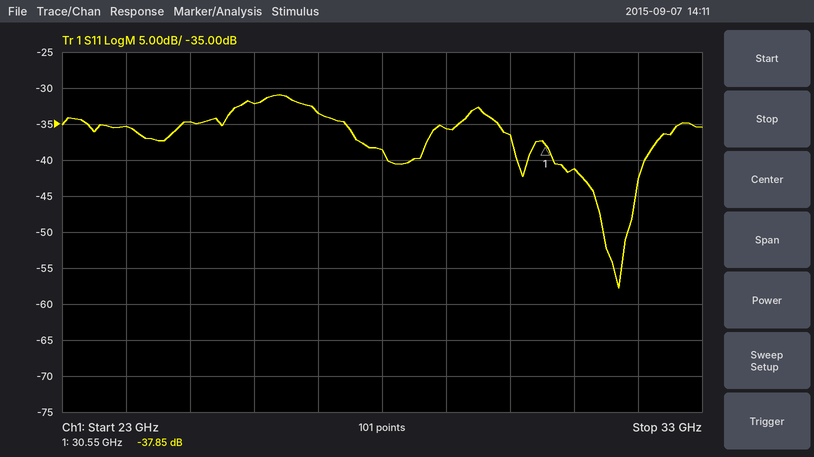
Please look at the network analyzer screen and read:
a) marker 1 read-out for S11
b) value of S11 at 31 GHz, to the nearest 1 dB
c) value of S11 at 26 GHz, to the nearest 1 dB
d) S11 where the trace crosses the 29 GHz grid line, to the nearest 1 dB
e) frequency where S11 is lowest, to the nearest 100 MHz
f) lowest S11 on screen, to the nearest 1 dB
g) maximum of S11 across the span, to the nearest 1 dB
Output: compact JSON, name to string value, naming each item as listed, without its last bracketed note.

{"marker 1 read-out for S11": "-37.85 dB", "value of S11 at 31 GHz, to the nearest 1 dB": "-41 dB", "value of S11 at 26 GHz, to the nearest 1 dB": "-32 dB", "S11 where the trace crosses the 29 GHz grid line, to the nearest 1 dB": "-36 dB", "frequency where S11 is lowest, to the nearest 100 MHz": "31.7 GHz", "lowest S11 on screen, to the nearest 1 dB": "-58 dB", "maximum of S11 across the span, to the nearest 1 dB": "-31 dB"}
